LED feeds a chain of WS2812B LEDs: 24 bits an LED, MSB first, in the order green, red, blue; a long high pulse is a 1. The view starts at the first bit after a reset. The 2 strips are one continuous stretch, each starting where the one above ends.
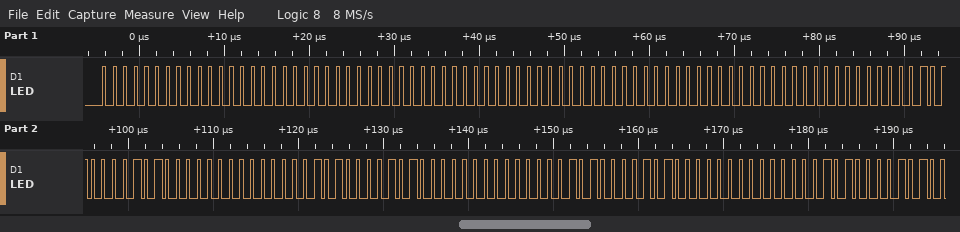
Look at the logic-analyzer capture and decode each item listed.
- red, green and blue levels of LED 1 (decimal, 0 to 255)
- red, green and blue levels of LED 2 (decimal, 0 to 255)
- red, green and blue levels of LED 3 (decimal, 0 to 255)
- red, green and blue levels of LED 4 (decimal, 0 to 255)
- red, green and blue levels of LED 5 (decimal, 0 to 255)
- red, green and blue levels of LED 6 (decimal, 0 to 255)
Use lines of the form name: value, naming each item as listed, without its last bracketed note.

red, green and blue levels of LED 1: 0, 0, 0
red, green and blue levels of LED 2: 0, 0, 0
red, green and blue levels of LED 3: 0, 0, 0
red, green and blue levels of LED 4: 10, 5, 0
red, green and blue levels of LED 5: 10, 5, 0
red, green and blue levels of LED 6: 10, 5, 0
